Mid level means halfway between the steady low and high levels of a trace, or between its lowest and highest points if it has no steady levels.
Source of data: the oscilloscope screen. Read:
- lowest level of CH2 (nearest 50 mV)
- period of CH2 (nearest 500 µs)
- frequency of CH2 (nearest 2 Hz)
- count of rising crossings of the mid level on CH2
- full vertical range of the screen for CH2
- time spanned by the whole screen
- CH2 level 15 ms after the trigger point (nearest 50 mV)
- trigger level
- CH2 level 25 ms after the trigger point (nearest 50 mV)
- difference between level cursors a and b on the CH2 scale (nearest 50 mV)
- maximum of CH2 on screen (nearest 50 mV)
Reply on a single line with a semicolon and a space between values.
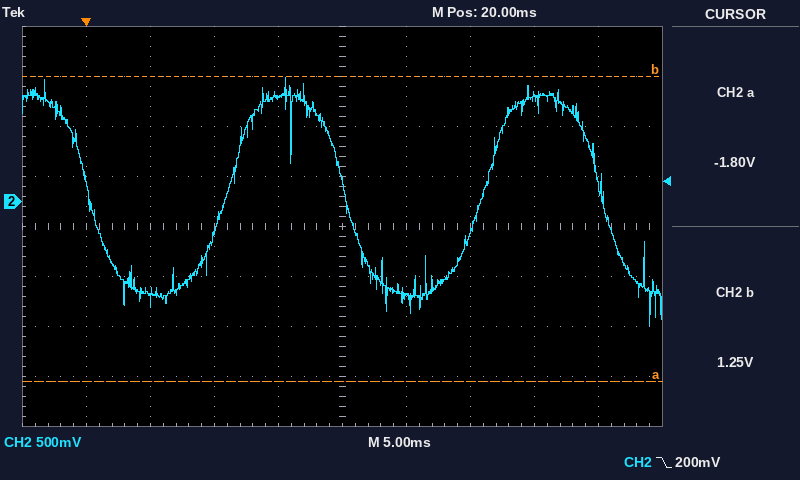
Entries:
-1.25 V; 20.0 ms; 50 Hz; 2; 4 V; 50 ms; 1.05 V; 200 mV; -950 mV; 3.05 V; 1.25 V
